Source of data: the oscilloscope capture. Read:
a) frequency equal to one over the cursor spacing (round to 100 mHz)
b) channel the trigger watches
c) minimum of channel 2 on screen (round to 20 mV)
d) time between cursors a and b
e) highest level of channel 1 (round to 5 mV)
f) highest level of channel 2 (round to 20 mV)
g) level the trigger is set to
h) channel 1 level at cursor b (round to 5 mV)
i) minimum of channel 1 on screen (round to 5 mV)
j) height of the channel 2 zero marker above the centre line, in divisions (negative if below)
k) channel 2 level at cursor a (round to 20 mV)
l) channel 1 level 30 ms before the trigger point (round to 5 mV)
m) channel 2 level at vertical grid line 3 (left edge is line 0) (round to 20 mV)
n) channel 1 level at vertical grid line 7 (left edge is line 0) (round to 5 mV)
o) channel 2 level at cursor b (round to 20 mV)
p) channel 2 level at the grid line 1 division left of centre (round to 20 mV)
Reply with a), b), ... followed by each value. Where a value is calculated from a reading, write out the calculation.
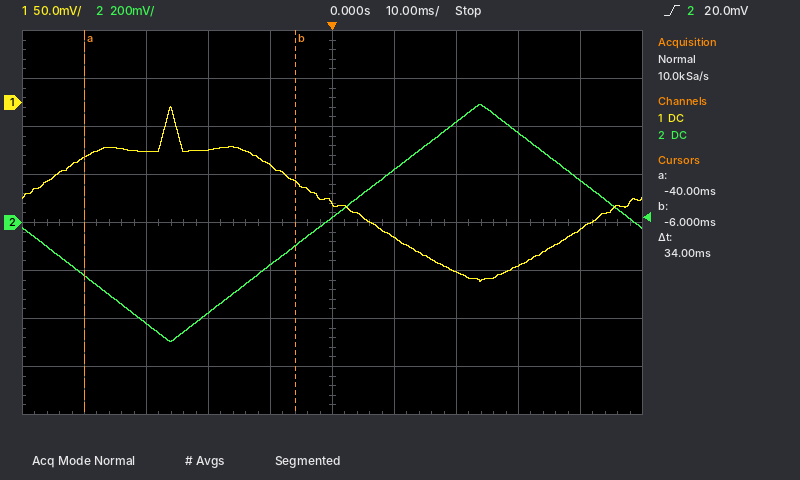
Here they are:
a) 1 / 34 ms ≈ 29.4 Hz
b) channel 2
c) -500 mV
d) 34 ms
e) -5 mV
f) 500 mV
g) 20.0 mV
h) -85 mV
i) -185 mV
j) 0.0 div
k) -220 mV
l) -50 mV
m) -380 mV
n) -175 mV
o) -100 mV
p) -180 mV
